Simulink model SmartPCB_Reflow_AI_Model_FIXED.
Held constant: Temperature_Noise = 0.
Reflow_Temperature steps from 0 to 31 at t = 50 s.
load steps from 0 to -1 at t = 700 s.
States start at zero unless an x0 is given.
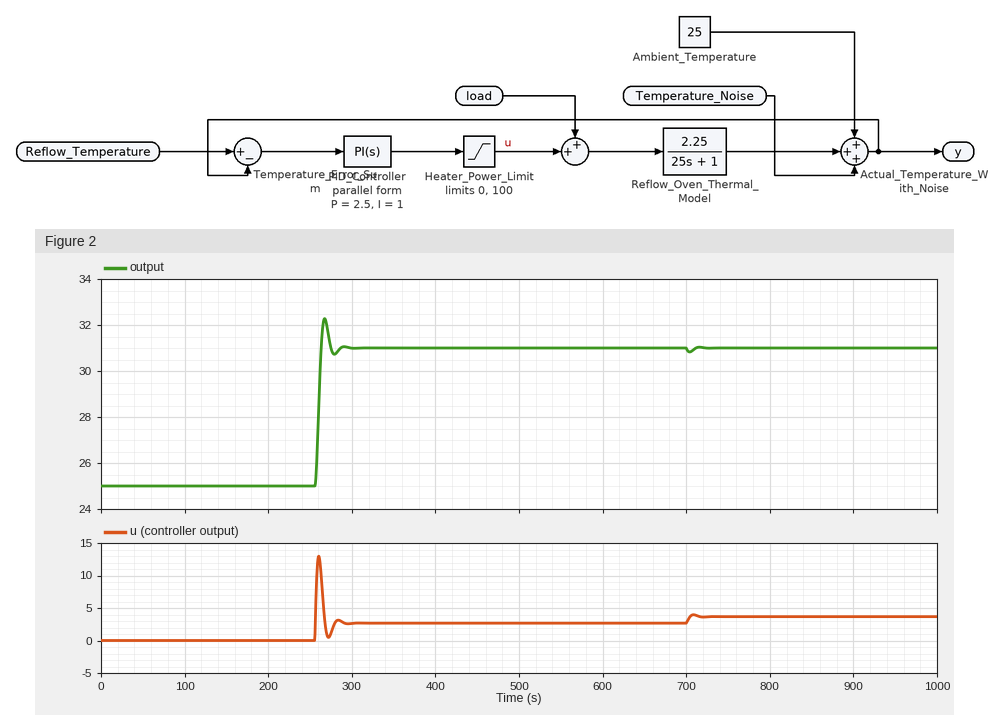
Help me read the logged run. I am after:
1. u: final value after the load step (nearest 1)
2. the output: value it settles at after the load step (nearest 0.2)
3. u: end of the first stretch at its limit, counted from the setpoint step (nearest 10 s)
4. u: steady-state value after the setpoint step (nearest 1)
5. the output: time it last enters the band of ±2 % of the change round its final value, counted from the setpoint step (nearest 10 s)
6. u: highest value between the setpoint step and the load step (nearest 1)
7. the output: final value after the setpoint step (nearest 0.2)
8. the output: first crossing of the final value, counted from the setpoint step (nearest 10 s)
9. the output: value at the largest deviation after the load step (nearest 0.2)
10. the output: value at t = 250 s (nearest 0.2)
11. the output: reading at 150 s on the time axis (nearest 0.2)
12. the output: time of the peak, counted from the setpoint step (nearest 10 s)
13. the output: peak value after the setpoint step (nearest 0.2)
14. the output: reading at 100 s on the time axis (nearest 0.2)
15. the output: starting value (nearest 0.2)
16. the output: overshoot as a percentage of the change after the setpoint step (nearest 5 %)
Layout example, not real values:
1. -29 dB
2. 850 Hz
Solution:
1. 4
2. 31.0
3. 210 s
4. 3
5. 230 s
6. 13
7. 31.0
8. 210 s
9. 30.8
10. 25.0
11. 25.0
12. 220 s
13. 32.2
14. 25.0
15. 25.0
16. 20 %
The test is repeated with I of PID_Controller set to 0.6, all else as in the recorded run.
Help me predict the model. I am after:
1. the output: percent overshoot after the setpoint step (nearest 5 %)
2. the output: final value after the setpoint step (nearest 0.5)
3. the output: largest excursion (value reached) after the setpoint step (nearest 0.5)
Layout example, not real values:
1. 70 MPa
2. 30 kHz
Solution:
1. 10 %
2. 31.0
3. 31.5
